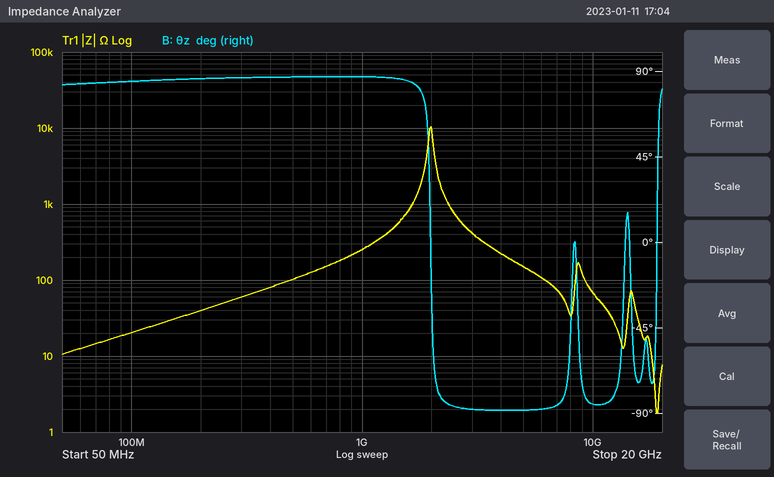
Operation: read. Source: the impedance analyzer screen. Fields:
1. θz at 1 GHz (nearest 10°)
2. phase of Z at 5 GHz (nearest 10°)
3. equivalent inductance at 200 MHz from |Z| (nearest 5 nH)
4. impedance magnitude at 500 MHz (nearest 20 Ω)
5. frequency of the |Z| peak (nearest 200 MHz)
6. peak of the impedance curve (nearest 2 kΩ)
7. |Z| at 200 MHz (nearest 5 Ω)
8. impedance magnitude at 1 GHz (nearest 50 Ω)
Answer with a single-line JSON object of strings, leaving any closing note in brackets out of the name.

{"θz at 1 GHz": "90°", "phase of Z at 5 GHz": "-90°", "equivalent inductance at 200 MHz from |Z|": "30 nH", "impedance magnitude at 500 MHz": "100 Ω", "frequency of the |Z| peak": "2.0 GHz", "peak of the impedance curve": "10 kΩ", "|Z| at 200 MHz": "40 Ω", "impedance magnitude at 1 GHz": "250 Ω"}
